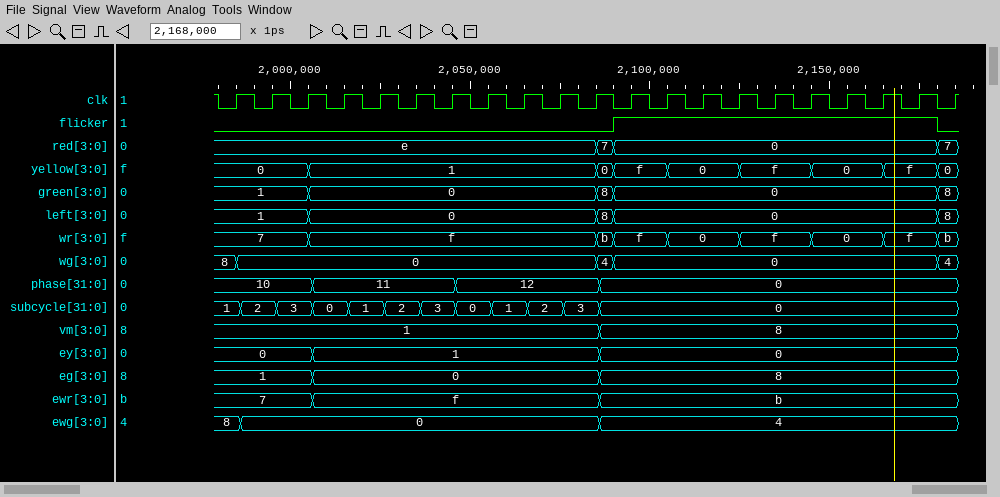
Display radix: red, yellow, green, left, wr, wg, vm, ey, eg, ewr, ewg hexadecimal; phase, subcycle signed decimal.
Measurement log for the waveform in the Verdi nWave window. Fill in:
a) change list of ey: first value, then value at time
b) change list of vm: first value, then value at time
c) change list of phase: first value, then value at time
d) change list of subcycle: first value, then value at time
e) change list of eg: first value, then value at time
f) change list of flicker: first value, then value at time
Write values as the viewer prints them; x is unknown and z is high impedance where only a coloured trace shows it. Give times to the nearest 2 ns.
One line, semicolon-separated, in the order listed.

0, 1 at 2006 ns, 0 at 2086 ns; 1, 8 at 2086 ns; 10, 11 at 2006 ns, 12 at 2046 ns, 0 at 2086 ns; 1, 2 at 1986 ns, 3 at 1996 ns, 0 at 2006 ns, 1 at 2016 ns, 2 at 2026 ns, 3 at 2036 ns, 0 at 2046 ns, 1 at 2056 ns, 2 at 2066 ns, 3 at 2076 ns, 0 at 2086 ns; 1, 0 at 2006 ns, 8 at 2086 ns; 0, 1 at 2090 ns, 0 at 2180 ns
